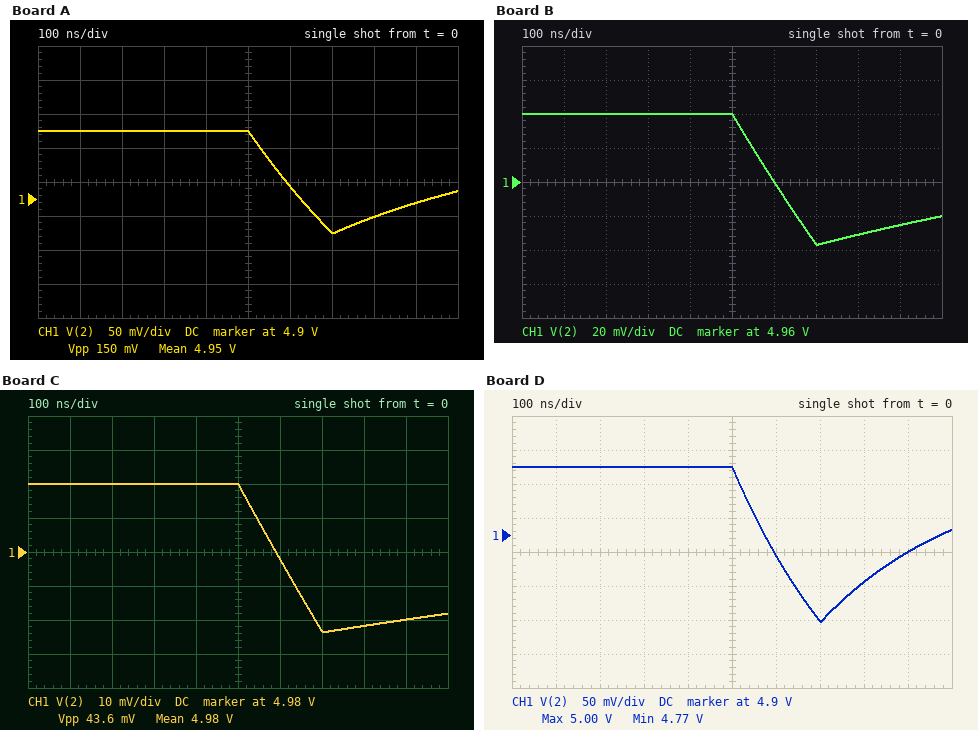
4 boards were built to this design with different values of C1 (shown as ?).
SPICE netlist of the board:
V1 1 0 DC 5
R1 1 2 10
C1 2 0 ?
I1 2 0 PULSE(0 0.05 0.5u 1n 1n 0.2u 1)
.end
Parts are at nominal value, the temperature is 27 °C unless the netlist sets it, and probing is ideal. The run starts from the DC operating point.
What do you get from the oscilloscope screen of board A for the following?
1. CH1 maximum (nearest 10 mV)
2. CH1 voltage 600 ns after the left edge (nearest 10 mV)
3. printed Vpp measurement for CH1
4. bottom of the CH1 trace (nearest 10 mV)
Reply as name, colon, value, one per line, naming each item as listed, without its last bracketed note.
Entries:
CH1 maximum: 5.00 V
CH1 voltage 600 ns after the left edge: 4.92 V
printed Vpp measurement for CH1: 150 mV
bottom of the CH1 trace: 4.85 V
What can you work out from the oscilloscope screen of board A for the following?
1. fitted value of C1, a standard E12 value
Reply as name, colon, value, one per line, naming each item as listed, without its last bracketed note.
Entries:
fitted value of C1, a standard E12 value: 56 nF
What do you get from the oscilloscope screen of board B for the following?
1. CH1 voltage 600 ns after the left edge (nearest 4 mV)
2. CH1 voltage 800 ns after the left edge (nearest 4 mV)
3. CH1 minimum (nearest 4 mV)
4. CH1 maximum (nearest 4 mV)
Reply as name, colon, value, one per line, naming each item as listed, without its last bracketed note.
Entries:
CH1 voltage 600 ns after the left edge: 4.960 V
CH1 voltage 800 ns after the left edge: 4.928 V
CH1 minimum: 4.924 V
CH1 maximum: 5.000 V
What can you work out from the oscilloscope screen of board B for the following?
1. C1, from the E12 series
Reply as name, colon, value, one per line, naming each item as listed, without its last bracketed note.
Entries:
C1, from the E12 series: 120 nF
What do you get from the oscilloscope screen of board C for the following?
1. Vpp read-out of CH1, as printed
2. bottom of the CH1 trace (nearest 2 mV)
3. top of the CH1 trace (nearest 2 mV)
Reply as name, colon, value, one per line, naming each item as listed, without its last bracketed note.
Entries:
Vpp read-out of CH1, as printed: 43.6 mV
bottom of the CH1 trace: 4.956 V
top of the CH1 trace: 5.000 V
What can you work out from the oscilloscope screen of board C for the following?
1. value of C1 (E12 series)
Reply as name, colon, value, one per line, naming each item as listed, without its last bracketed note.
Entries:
value of C1: 220 nF
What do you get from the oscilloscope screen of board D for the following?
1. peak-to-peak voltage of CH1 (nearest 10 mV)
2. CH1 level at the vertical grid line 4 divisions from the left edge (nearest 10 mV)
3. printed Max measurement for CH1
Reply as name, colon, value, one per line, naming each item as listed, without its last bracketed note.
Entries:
peak-to-peak voltage of CH1: 230 mV
CH1 level at the vertical grid line 4 divisions from the left edge: 5.00 V
printed Max measurement for CH1: 5.00 V
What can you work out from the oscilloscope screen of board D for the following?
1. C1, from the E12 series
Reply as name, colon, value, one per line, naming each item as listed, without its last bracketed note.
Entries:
C1, from the E12 series: 33 nF
